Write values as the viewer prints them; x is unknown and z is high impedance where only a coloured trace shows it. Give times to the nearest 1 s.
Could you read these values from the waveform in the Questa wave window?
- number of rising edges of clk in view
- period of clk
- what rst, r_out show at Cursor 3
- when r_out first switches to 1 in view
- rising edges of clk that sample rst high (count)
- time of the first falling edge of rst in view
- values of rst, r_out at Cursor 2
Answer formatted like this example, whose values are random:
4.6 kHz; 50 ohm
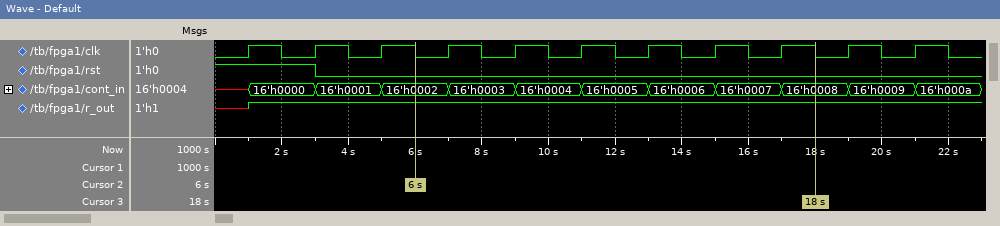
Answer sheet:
11; 2 s; rst=0, r_out=1; 1 s; 2; 3 s; rst=0, r_out=1
